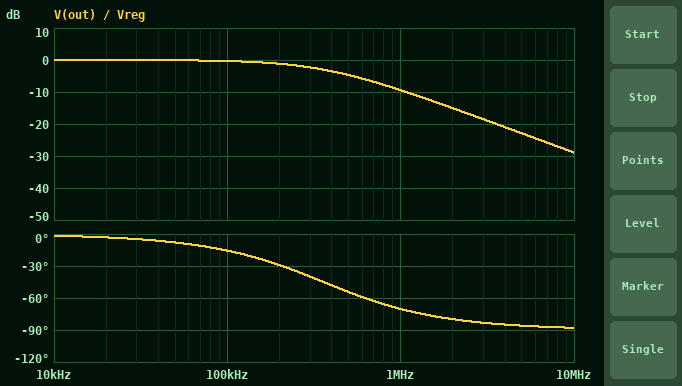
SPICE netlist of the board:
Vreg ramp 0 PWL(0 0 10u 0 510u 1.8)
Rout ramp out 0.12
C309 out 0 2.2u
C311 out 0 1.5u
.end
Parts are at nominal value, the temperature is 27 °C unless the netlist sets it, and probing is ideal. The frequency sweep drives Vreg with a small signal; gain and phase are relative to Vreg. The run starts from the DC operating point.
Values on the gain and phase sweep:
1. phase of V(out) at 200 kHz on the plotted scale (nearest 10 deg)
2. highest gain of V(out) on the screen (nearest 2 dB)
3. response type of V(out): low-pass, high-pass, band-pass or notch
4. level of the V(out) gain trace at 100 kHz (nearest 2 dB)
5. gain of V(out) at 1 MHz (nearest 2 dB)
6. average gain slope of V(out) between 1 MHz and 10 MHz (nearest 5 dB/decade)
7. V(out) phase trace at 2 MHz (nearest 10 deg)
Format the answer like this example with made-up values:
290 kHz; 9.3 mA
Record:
-30 deg; 0 dB; low-pass; 0 dB; -10 dB; -20 dB/decade; -80 deg
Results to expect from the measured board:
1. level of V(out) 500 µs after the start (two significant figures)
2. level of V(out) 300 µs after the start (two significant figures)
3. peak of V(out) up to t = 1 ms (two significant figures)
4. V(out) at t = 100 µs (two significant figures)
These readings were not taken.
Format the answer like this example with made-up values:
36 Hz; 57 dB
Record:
1.8 V; 1.0 V; 1.8 V; 320 mV
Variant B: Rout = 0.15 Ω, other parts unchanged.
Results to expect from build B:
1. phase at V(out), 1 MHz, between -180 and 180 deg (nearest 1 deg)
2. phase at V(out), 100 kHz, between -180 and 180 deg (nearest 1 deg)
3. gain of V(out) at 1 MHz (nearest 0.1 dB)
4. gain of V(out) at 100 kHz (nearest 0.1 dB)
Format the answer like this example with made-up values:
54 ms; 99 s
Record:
-74 deg; -19 deg; -11.2 dB; -0.5 dB
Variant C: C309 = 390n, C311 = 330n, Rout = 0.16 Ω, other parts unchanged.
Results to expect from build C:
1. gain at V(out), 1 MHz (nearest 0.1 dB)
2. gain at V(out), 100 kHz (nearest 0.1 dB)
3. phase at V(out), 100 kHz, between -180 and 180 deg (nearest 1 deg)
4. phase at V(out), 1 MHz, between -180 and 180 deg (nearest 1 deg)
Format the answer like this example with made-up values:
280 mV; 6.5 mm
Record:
-1.8 dB; 0 dB; -4 deg; -36 deg
